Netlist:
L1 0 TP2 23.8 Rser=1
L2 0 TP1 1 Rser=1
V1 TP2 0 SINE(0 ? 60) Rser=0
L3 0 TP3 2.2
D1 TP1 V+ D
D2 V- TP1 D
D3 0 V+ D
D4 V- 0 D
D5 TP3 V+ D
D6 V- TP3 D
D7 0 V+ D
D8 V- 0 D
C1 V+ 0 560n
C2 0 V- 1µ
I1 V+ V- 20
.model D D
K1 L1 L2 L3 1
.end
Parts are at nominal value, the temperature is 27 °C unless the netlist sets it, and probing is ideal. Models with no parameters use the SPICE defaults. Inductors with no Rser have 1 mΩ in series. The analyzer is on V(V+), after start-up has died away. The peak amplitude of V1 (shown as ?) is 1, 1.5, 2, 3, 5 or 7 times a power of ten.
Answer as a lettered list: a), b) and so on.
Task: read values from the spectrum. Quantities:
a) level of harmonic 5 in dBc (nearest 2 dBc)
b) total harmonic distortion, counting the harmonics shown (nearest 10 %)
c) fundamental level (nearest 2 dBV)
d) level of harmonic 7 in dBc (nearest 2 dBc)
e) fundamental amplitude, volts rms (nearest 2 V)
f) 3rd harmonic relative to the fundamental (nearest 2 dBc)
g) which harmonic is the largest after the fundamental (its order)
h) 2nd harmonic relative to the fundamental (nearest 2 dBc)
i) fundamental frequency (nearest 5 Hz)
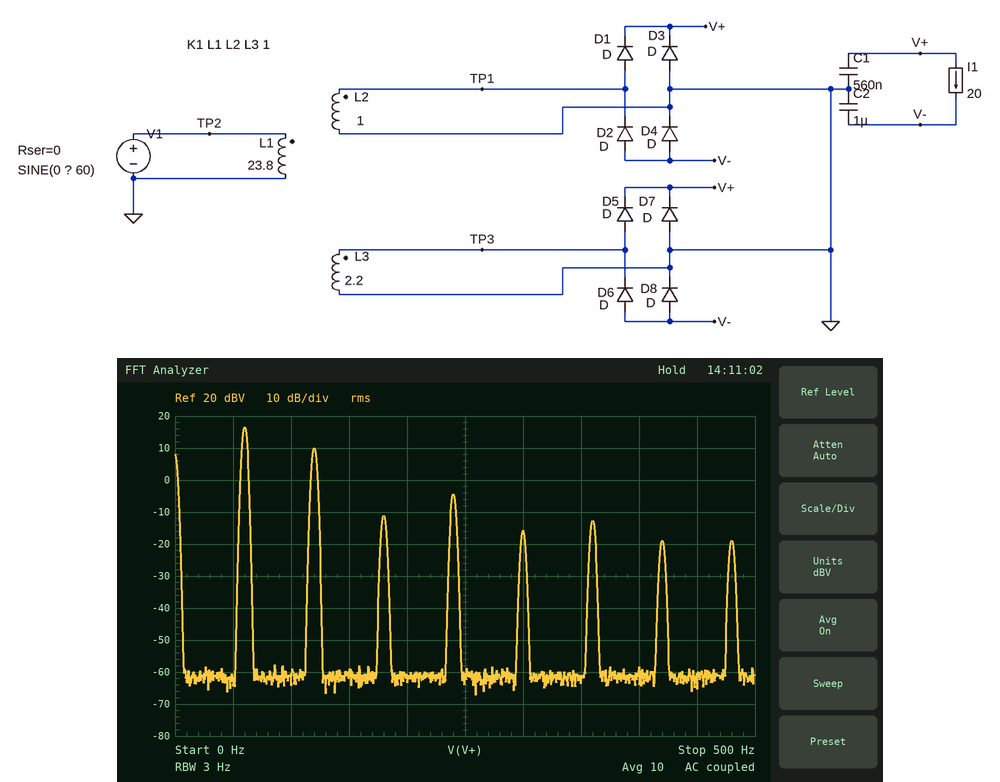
a) -32 dBc
b) 50 %
c) 16 dBV
d) -36 dBc
e) 6 V
f) -28 dBc
g) 2
h) -6 dBc
i) 60 Hz
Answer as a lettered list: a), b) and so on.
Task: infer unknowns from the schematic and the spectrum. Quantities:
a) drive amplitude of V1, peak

a) 70 V
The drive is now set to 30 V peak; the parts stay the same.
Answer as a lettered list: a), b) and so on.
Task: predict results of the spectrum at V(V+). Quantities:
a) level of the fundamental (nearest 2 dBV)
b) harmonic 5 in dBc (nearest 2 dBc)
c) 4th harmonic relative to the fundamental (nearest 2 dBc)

a) 8 dBV
b) -24 dBc
c) -22 dBc
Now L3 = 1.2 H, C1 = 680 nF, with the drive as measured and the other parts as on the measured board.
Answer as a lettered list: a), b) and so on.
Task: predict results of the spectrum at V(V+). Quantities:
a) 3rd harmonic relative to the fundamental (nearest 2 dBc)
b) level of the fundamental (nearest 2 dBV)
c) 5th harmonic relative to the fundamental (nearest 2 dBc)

a) -30 dBc
b) 14 dBV
c) -34 dBc
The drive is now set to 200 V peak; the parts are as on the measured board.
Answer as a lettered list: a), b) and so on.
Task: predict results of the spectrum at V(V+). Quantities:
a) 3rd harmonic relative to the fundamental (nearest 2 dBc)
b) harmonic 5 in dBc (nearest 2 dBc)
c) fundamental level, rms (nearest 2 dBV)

a) -38 dBc
b) -42 dBc
c) 26 dBV
